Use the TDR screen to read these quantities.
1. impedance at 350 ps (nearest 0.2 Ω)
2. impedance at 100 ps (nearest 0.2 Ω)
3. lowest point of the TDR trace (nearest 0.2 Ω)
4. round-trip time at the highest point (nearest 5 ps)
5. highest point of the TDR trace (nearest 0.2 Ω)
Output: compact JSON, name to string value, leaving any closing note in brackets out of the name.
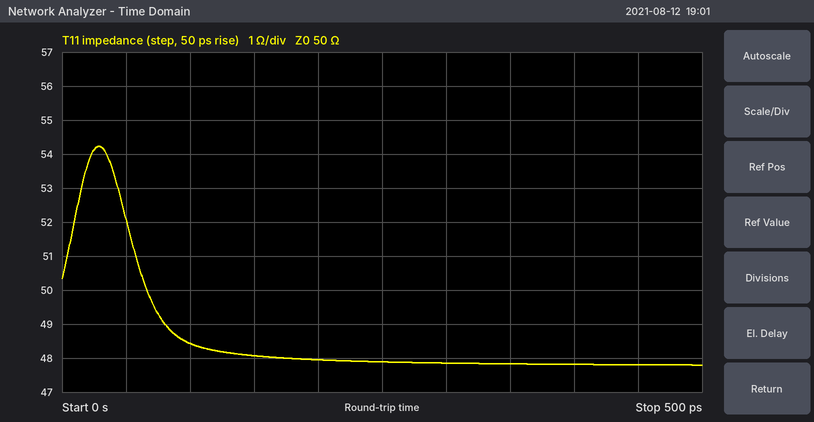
{"impedance at 350 ps": "47.8 Ω", "impedance at 100 ps": "48.4 Ω", "lowest point of the TDR trace": "47.8 Ω", "round-trip time at the highest point": "30 ps", "highest point of the TDR trace": "54.2 Ω"}
